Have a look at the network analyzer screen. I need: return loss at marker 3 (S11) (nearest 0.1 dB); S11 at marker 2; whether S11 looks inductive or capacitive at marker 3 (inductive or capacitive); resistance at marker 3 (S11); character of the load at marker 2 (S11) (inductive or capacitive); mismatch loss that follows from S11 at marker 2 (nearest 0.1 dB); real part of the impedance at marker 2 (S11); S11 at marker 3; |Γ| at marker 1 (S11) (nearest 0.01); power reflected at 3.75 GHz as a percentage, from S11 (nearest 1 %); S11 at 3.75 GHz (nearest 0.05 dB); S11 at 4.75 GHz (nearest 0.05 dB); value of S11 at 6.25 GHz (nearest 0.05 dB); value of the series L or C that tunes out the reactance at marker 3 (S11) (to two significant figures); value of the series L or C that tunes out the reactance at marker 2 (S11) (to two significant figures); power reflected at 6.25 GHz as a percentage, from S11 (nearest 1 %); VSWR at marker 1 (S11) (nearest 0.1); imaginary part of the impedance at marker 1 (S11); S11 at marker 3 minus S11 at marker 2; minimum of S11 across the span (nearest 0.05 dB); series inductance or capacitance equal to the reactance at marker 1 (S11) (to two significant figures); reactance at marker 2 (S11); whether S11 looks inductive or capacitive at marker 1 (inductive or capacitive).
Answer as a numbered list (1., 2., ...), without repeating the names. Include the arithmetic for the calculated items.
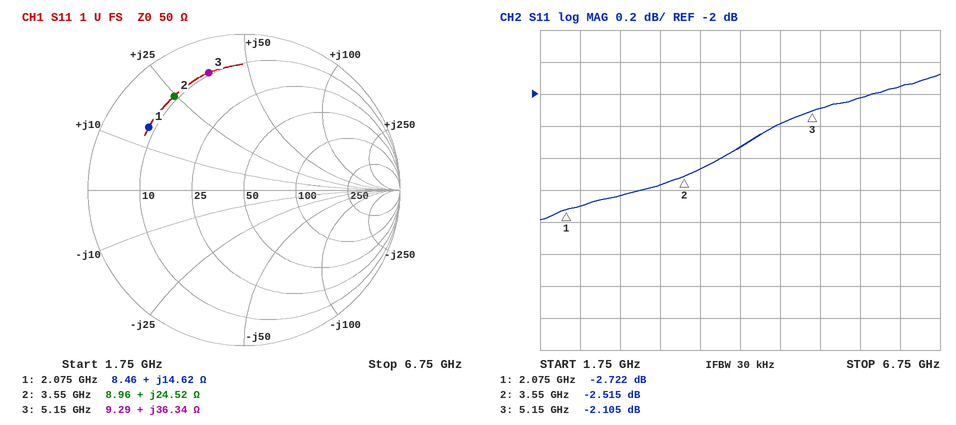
1. 2.1 dB
2. -2.515 dB
3. inductive
4. 9.29 Ω
5. inductive
6. −10 log10(1 − 10^(-2.515/10)) ≈ 3.6 dB
7. 8.96 Ω
8. -2.105 dB
9. 0.73
10. 10^(-2.45/10) ≈ 57 %
11. -2.45 dB
12. -2.20 dB
13. -1.95 dB
14. C = 1/(2π × 5.15 GHz × 36.34 Ω) ≈ 850 fF
15. C = 1/(2π × 3.55 GHz × 24.52 Ω) ≈ 1.8 pF
16. 10^(-1.95/10) ≈ 64 %
17. (1 + 0.7310)/(1 − 0.7310) ≈ 6.4
18. +14.62 Ω
19. -2.105 − (-2.515) = 0.410 dB
20. -2.80 dB
21. L = 14.62 Ω/(2π × 2.075 GHz) ≈ 1.1 nH
22. +24.52 Ω
23. inductive
